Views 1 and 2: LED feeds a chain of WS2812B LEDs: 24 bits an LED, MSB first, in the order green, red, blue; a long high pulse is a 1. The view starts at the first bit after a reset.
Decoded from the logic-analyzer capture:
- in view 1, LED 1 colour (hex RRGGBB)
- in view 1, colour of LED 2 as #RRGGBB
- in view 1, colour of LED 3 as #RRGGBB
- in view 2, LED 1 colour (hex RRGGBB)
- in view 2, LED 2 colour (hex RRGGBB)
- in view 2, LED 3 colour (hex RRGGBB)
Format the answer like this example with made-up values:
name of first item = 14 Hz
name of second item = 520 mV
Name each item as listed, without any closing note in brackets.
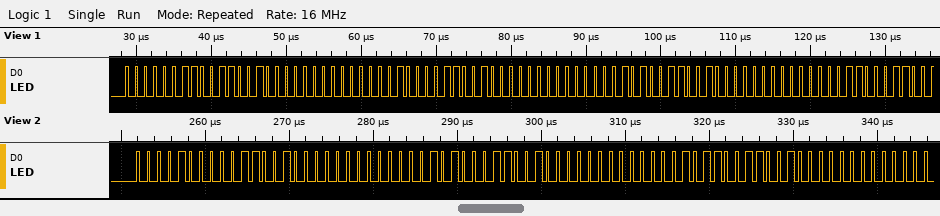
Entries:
in view 1, LED 1 colour = #320300
in view 1, colour of LED 2 as #RRGGBB = #320400
in view 1, colour of LED 3 as #RRGGBB = #320500
in view 2, LED 1 colour = #320800
in view 2, LED 2 colour = #320A00
in view 2, LED 3 colour = #320B00
